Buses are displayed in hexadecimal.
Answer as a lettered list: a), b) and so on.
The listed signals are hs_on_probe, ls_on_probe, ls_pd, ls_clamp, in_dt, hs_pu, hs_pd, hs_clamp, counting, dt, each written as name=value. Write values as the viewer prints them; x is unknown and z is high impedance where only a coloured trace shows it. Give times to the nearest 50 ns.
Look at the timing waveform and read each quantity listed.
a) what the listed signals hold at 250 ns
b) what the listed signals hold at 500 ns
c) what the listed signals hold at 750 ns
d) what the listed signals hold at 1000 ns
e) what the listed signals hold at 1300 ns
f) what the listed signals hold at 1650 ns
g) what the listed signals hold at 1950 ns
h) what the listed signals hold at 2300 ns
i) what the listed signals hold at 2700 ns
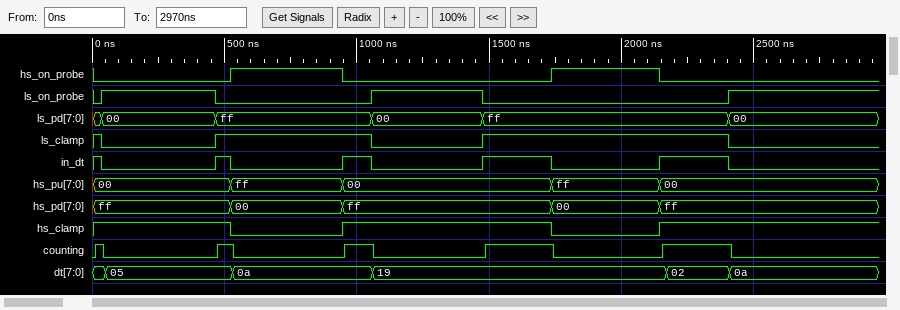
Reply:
a) hs_on_probe=0, ls_on_probe=1, ls_pd=00, ls_clamp=0, in_dt=0, hs_pu=00, hs_pd=ff, hs_clamp=1, counting=0, dt=05
b) hs_on_probe=0, ls_on_probe=0, ls_pd=ff, ls_clamp=1, in_dt=1, hs_pu=00, hs_pd=ff, hs_clamp=1, counting=1, dt=05
c) hs_on_probe=1, ls_on_probe=0, ls_pd=ff, ls_clamp=1, in_dt=0, hs_pu=ff, hs_pd=00, hs_clamp=0, counting=0, dt=0a
d) hs_on_probe=0, ls_on_probe=0, ls_pd=ff, ls_clamp=1, in_dt=1, hs_pu=00, hs_pd=ff, hs_clamp=1, counting=1, dt=0a
e) hs_on_probe=0, ls_on_probe=1, ls_pd=00, ls_clamp=0, in_dt=0, hs_pu=00, hs_pd=ff, hs_clamp=1, counting=0, dt=19
f) hs_on_probe=0, ls_on_probe=0, ls_pd=ff, ls_clamp=1, in_dt=1, hs_pu=00, hs_pd=ff, hs_clamp=1, counting=1, dt=19
g) hs_on_probe=1, ls_on_probe=0, ls_pd=ff, ls_clamp=1, in_dt=0, hs_pu=ff, hs_pd=00, hs_clamp=0, counting=0, dt=19
h) hs_on_probe=0, ls_on_probe=0, ls_pd=ff, ls_clamp=1, in_dt=1, hs_pu=00, hs_pd=ff, hs_clamp=1, counting=1, dt=02
i) hs_on_probe=0, ls_on_probe=1, ls_pd=00, ls_clamp=0, in_dt=0, hs_pu=00, hs_pd=ff, hs_clamp=1, counting=0, dt=0a
